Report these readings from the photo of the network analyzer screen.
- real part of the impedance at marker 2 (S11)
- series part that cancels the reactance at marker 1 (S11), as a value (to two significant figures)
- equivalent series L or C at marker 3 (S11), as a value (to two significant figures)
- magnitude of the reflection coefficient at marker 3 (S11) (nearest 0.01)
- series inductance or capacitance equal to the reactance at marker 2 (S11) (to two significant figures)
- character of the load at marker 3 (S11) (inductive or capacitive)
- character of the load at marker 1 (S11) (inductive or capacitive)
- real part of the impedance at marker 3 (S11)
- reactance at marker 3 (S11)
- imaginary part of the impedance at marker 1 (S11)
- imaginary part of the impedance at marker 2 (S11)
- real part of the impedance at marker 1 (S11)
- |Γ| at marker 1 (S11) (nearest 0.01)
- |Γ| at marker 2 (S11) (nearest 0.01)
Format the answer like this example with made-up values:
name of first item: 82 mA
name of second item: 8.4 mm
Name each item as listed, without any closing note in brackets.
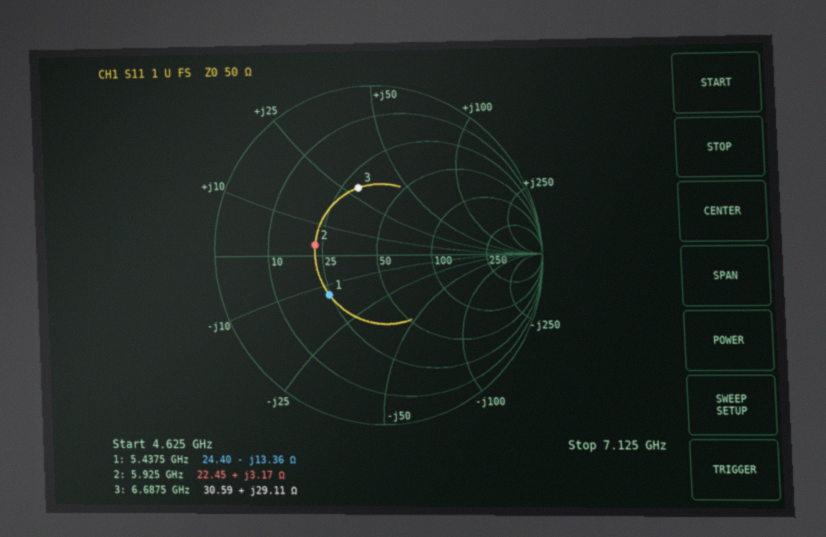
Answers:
real part of the impedance at marker 2: 22.45 Ω
series part that cancels the reactance at marker 1 (S11), as a value: 390 pH
equivalent series L or C at marker 3 (S11), as a value: 690 pH
magnitude of the reflection coefficient at marker 3 (S11): 0.41
series inductance or capacitance equal to the reactance at marker 2 (S11): 85 pH
character of the load at marker 3 (S11): inductive
character of the load at marker 1 (S11): capacitive
real part of the impedance at marker 3: 30.59 Ω
reactance at marker 3: +29.11 Ω
imaginary part of the impedance at marker 1: -13.36 Ω
imaginary part of the impedance at marker 2: +3.17 Ω
real part of the impedance at marker 1: 24.40 Ω
|Γ| at marker 1 (S11): 0.38
|Γ| at marker 2 (S11): 0.38
